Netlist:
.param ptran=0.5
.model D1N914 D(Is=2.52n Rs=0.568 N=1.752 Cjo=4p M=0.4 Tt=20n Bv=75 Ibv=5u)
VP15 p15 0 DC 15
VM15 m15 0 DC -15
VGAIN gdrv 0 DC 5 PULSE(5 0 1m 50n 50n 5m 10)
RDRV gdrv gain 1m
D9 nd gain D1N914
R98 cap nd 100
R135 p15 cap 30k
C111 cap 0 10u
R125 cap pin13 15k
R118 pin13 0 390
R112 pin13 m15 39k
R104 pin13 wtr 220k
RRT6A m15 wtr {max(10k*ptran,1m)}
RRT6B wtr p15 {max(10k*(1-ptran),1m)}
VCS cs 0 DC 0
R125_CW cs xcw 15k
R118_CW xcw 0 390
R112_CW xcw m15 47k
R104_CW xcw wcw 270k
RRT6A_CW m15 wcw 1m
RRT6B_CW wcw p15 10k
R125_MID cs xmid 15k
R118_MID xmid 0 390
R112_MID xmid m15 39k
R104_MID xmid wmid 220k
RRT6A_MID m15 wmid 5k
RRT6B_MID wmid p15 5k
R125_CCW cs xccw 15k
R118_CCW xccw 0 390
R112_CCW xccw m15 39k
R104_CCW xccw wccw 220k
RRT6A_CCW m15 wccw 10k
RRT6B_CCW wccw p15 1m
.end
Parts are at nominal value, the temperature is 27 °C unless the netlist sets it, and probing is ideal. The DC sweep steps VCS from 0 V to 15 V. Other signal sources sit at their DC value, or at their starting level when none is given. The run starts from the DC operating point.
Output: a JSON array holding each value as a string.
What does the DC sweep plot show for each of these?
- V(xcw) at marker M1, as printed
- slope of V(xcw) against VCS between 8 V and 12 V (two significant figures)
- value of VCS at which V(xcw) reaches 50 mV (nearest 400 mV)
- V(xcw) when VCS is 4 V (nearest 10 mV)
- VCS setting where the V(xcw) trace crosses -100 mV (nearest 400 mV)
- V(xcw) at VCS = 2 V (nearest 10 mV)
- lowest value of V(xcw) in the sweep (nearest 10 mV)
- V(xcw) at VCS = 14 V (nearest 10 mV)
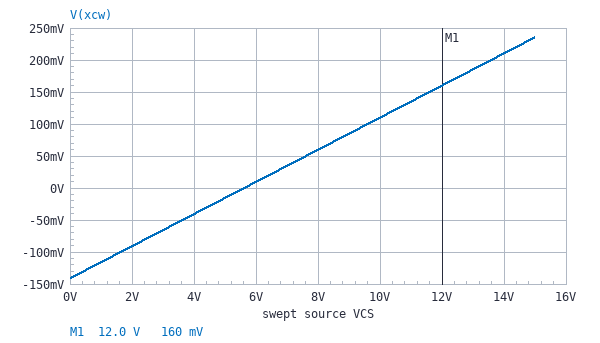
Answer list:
["160 mV", "0.025 V/V", "7.6 V", "-40 mV", "1.6 V", "-90 mV", "-140 mV", "210 mV"]
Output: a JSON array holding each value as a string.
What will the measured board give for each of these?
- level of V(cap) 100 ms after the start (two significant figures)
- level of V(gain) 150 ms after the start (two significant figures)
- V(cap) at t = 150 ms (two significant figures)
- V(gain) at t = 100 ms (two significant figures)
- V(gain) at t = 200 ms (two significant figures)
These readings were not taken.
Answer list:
["3.3 V", "5.0 V", "3.9 V", "5.0 V", "5.0 V"]
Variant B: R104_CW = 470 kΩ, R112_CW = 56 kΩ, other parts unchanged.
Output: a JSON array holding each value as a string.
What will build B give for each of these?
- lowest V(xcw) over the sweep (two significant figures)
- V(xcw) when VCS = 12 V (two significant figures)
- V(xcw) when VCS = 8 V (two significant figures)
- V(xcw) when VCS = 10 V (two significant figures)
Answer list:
["-110 mV", "190 mV", "88 mV", "140 mV"]
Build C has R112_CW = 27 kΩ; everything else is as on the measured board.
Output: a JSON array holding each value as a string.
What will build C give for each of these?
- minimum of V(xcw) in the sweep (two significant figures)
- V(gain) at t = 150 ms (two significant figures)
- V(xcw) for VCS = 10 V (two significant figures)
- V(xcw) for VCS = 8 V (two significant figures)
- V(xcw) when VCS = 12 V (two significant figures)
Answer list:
["-230 mV", "5.0 V", "21 mV", "-29 mV", "71 mV"]
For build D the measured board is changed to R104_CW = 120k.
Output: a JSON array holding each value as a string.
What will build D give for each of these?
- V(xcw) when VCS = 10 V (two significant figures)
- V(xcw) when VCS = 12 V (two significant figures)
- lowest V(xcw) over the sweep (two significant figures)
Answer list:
["84 mV", "130 mV", "-170 mV"]
